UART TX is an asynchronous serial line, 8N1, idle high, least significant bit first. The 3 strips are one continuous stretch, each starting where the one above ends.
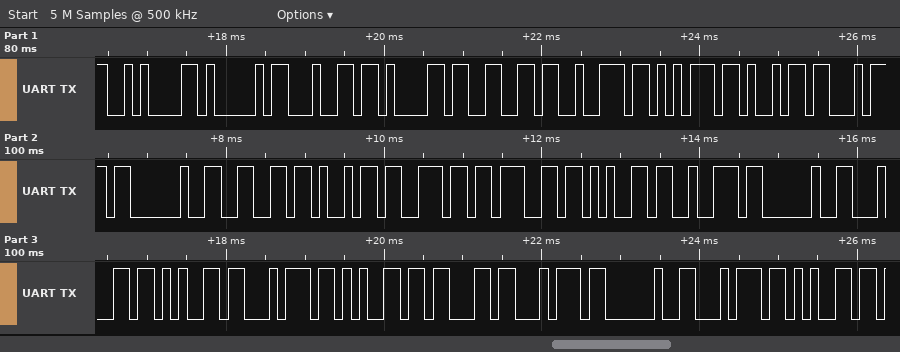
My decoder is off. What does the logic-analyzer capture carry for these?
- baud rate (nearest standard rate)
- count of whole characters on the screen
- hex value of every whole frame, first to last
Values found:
9600 baud
26
0A 41 64 61 66 72 75 69 74 20 66 69 6E 67 65 72 20 64 65 74 65 63 74 20 74 65
